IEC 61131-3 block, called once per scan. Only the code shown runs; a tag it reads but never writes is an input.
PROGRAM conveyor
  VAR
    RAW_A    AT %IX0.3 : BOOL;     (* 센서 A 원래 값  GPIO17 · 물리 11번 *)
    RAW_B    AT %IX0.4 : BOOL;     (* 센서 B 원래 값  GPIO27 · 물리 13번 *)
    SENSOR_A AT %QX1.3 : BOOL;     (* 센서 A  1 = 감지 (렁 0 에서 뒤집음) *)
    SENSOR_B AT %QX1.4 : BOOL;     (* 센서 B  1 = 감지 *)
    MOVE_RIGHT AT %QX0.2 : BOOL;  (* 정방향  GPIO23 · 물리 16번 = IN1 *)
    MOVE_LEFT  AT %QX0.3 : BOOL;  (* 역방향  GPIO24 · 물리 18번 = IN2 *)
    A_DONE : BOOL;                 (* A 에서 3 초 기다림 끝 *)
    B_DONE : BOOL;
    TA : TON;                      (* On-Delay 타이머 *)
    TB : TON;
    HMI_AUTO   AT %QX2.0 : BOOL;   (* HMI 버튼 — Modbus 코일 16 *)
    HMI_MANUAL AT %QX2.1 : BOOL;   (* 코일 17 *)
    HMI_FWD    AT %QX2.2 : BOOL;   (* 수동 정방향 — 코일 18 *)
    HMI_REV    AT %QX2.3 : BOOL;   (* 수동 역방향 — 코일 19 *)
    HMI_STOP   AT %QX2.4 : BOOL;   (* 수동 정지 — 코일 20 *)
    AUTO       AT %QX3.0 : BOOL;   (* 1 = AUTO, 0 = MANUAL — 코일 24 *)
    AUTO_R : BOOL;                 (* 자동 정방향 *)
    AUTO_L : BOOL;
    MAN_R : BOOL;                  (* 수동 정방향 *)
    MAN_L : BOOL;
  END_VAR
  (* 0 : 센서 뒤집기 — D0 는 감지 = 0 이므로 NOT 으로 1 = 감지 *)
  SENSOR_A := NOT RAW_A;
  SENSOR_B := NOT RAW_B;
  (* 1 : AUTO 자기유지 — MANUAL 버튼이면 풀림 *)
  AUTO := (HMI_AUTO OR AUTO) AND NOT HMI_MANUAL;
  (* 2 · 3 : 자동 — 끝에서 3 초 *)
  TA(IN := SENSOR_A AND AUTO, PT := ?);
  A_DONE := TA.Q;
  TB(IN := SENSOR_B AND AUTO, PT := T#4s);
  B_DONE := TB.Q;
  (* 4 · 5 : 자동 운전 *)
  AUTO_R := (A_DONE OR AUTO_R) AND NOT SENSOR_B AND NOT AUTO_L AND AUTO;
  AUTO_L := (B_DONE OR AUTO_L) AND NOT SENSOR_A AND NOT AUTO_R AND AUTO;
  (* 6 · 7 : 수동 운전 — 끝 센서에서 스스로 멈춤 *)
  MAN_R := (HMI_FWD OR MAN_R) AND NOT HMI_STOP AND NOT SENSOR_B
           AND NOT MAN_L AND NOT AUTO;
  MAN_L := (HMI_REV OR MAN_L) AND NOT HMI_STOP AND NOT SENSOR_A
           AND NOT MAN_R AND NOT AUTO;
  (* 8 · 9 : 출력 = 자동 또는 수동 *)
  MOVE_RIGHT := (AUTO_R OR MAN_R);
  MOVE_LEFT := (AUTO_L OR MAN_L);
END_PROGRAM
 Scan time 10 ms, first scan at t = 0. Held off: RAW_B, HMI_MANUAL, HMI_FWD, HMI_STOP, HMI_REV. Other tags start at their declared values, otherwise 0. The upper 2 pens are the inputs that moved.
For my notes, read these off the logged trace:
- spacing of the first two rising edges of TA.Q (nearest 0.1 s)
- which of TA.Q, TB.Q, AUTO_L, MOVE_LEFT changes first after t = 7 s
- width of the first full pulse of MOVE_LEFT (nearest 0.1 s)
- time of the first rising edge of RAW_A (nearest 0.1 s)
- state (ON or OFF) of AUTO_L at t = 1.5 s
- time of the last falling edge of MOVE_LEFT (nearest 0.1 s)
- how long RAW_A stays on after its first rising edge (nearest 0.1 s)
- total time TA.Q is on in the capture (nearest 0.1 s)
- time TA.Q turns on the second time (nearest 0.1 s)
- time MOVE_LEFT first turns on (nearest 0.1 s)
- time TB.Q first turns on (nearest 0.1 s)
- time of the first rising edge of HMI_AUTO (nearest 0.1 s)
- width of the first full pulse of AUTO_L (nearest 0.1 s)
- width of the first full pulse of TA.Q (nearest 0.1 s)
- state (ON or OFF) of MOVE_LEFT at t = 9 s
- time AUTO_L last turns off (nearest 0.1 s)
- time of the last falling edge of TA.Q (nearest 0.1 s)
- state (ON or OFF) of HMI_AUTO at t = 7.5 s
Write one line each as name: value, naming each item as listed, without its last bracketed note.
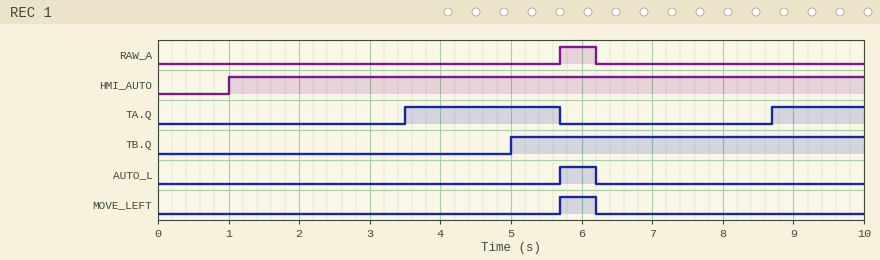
spacing of the first two rising edges of TA.Q: 5.2 s
which of TA.Q, TB.Q, AUTO_L, MOVE_LEFT changes first after t = 7 s: TA.Q
width of the first full pulse of MOVE_LEFT: 0.5 s
time of the first rising edge of RAW_A: 5.7 s
state (ON or OFF) of AUTO_L at t = 1.5 s: OFF
time of the last falling edge of MOVE_LEFT: 6.2 s
how long RAW_A stays on after its first rising edge: 0.5 s
total time TA.Q is on in the capture: 3.5 s
time TA.Q turns on the second time: 8.7 s
time MOVE_LEFT first turns on: 5.7 s
time TB.Q first turns on: 5.0 s
time of the first rising edge of HMI_AUTO: 1.0 s
width of the first full pulse of AUTO_L: 0.5 s
width of the first full pulse of TA.Q: 2.2 s
state (ON or OFF) of MOVE_LEFT at t = 9 s: OFF
time AUTO_L last turns off: 6.2 s
time of the last falling edge of TA.Q: 5.7 s
state (ON or OFF) of HMI_AUTO at t = 7.5 s: ON
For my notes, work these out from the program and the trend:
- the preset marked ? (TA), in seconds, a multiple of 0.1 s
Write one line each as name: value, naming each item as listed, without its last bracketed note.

the preset marked ? (TA), in seconds, a multiple of 0.1 s: 2.5 s
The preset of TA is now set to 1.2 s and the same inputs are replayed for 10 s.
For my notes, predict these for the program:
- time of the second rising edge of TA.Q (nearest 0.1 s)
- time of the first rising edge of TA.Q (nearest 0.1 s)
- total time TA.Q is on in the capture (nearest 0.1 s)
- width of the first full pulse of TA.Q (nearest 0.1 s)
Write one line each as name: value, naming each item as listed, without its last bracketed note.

time of the second rising edge of TA.Q: 7.4 s
time of the first rising edge of TA.Q: 2.2 s
total time TA.Q is on in the capture: 6.1 s
width of the first full pulse of TA.Q: 3.5 s
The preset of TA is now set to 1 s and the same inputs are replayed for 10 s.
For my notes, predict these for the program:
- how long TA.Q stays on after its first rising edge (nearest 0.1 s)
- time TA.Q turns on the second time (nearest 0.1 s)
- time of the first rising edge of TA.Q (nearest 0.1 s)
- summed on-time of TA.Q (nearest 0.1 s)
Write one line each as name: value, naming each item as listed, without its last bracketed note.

how long TA.Q stays on after its first rising edge: 3.7 s
time TA.Q turns on the second time: 7.2 s
time of the first rising edge of TA.Q: 2.0 s
summed on-time of TA.Q: 6.5 s
